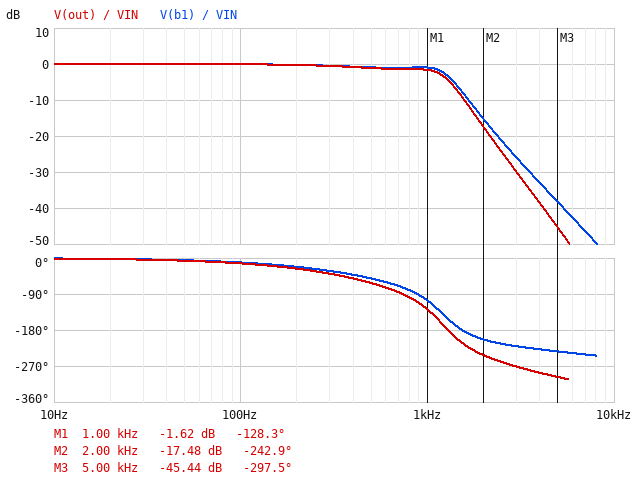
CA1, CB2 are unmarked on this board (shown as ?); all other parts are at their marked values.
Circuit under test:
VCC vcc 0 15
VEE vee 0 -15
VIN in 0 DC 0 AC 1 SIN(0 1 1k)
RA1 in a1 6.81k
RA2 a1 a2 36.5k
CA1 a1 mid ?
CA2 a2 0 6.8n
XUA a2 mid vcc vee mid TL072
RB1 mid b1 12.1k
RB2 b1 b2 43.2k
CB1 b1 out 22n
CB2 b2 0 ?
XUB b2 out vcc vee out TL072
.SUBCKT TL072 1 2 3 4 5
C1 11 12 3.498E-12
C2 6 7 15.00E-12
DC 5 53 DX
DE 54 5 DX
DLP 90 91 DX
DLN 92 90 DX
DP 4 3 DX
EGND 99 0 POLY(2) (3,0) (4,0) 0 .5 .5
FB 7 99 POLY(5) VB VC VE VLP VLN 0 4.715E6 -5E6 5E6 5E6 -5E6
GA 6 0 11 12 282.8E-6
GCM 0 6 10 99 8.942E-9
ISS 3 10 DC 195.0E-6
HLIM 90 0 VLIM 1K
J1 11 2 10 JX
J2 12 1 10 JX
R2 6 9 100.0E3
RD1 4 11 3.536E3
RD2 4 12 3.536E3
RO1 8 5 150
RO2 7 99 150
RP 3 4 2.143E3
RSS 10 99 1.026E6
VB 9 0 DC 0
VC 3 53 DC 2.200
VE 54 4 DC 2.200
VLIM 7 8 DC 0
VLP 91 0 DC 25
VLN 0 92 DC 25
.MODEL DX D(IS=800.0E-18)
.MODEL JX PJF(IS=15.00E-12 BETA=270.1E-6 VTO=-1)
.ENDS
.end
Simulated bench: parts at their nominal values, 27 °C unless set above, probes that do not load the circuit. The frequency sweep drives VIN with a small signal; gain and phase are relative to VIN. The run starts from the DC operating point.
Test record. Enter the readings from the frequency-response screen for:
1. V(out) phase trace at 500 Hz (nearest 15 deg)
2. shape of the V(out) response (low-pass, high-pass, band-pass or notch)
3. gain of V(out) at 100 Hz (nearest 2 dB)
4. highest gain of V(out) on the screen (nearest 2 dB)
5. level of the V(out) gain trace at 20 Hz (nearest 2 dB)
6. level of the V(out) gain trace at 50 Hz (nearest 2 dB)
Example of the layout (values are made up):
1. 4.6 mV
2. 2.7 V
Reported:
1. -60 deg
2. low-pass
3. 0 dB
4. 0 dB
5. 0 dB
6. 0 dB
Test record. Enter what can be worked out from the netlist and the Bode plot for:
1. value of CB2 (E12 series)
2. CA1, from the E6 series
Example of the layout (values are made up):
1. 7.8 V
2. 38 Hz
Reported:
1. 1.5 nF
2. 4.7 nF
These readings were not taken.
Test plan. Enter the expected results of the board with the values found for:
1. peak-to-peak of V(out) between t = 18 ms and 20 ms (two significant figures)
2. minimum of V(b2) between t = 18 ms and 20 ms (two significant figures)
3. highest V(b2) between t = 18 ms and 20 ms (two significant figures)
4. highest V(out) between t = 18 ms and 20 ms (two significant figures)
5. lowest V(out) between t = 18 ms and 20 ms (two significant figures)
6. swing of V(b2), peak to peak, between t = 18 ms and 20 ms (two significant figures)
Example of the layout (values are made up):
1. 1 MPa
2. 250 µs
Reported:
1. 1.7 V
2. -830 mV
3. 830 mV
4. 830 mV
5. -830 mV
6. 1.7 V
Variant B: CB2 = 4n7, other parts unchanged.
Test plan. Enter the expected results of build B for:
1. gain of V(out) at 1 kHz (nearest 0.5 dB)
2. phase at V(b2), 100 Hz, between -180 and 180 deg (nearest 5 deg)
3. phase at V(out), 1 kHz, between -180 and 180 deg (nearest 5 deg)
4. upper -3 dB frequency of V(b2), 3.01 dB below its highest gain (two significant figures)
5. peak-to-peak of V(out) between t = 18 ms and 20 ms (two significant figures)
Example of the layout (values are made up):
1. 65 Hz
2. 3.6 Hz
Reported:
1. -12.0 dB
2. -20 deg
3. 165 deg
4. 590 Hz
5. 510 mV
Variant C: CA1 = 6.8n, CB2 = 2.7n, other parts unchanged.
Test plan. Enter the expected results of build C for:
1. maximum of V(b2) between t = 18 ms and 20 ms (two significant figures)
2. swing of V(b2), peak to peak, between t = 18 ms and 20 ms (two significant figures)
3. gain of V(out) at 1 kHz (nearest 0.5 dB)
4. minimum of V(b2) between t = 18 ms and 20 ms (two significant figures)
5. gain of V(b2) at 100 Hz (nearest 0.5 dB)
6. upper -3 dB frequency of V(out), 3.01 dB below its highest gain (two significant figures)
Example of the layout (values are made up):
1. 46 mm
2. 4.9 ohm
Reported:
1. 540 mV
2. 1.1 V
3. -5.5 dB
4. -540 mV
5. 0 dB
6. 870 Hz
